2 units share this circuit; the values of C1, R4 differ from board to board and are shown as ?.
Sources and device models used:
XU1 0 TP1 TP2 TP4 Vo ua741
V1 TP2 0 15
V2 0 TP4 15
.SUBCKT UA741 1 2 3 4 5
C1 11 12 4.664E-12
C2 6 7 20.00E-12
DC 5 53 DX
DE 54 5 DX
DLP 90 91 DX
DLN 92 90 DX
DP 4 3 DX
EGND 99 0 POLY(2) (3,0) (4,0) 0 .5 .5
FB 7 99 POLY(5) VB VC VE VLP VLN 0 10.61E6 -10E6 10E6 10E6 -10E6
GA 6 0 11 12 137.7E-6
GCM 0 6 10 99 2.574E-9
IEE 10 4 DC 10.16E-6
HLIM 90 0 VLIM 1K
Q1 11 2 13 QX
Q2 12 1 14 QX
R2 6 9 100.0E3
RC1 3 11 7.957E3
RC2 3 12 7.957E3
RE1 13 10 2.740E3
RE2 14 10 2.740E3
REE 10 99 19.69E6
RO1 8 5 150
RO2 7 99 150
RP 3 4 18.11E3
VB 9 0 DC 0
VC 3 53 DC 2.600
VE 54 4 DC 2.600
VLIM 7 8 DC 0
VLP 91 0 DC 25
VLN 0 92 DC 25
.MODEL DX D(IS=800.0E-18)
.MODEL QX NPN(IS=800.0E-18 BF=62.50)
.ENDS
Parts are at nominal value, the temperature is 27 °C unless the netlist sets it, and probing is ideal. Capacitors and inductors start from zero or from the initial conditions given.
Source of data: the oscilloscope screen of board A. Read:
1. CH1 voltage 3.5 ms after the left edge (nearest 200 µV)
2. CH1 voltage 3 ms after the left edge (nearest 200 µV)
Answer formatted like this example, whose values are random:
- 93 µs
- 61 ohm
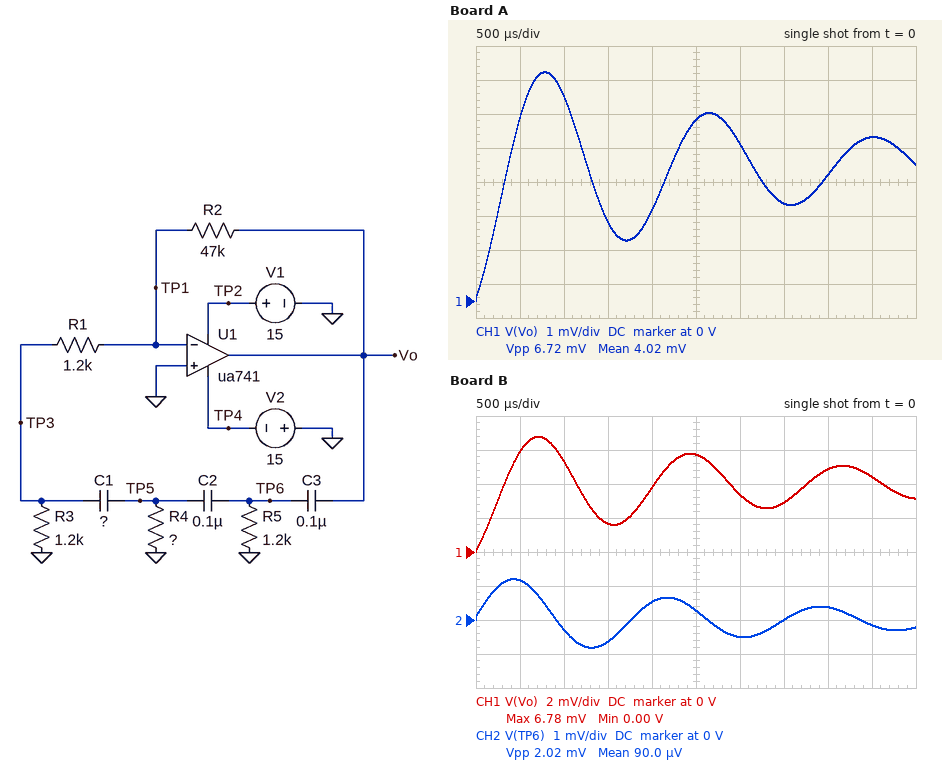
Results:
- 2.8 mV
- 4.6 mV
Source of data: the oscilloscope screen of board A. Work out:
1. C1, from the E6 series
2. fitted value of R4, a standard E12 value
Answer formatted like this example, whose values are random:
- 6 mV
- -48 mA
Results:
- 68 nF
- 3.9 kΩ
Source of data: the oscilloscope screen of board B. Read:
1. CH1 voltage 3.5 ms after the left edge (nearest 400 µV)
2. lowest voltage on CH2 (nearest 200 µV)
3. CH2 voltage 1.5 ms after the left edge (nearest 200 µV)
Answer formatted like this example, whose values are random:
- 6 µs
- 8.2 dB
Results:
- 2.8 mV
- -800 µV
- -600 µV
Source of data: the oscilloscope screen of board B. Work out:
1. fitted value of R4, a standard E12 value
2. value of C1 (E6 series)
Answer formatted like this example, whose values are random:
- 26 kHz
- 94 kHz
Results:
- 470 Ω
- 330 nF
